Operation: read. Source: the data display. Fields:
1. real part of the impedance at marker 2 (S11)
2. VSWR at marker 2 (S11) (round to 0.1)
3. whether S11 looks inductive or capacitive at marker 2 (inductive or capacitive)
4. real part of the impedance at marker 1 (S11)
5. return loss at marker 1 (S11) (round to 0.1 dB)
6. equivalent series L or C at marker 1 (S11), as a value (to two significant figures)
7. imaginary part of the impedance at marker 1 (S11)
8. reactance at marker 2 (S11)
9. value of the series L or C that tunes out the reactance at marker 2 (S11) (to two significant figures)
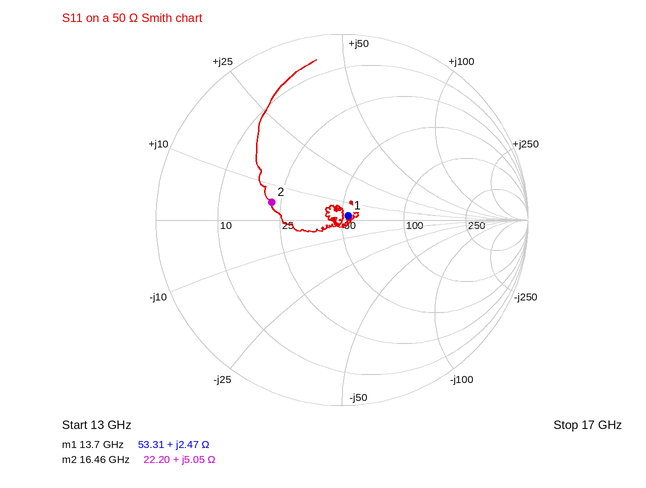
22.20 Ω
2.3
inductive
53.31 Ω
28.0 dB
29 pH
+2.47 Ω
+5.05 Ω
1.9 pF
